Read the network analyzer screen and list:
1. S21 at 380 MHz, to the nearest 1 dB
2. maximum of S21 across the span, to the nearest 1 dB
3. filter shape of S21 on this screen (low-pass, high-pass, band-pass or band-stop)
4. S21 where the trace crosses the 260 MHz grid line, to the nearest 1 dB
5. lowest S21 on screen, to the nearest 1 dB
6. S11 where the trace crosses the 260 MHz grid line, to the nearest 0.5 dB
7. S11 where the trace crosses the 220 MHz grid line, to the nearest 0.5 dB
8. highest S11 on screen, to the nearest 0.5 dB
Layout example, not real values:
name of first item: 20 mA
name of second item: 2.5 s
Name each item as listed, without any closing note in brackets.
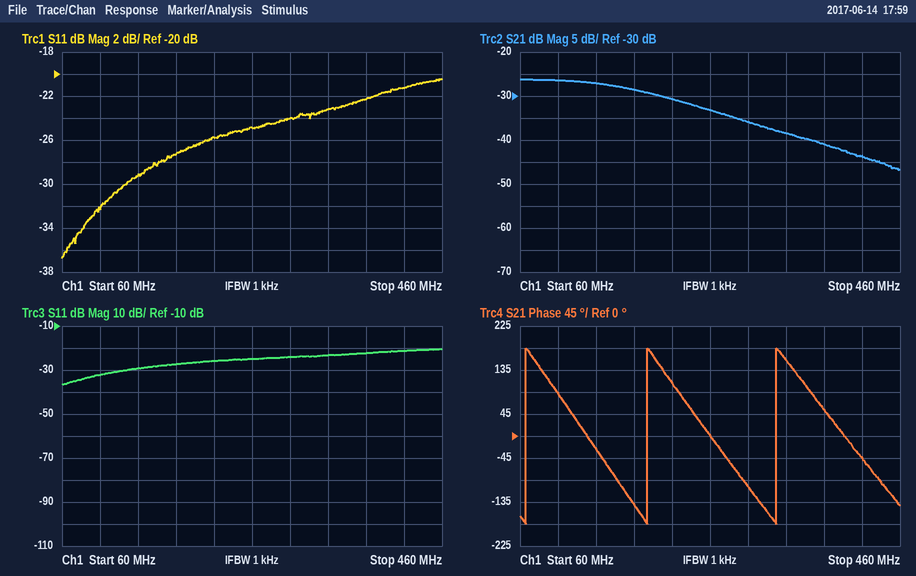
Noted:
S21 at 380 MHz, to the nearest 1 dB: -41 dB
maximum of S21 across the span, to the nearest 1 dB: -26 dB
filter shape of S21 on this screen: low-pass
S21 where the trace crosses the 260 MHz grid line, to the nearest 1 dB: -33 dB
lowest S21 on screen, to the nearest 1 dB: -47 dB
S11 where the trace crosses the 260 MHz grid line, to the nearest 0.5 dB: -25.0 dB
S11 where the trace crosses the 220 MHz grid line, to the nearest 0.5 dB: -26.0 dB
highest S11 on screen, to the nearest 0.5 dB: -20.5 dB
